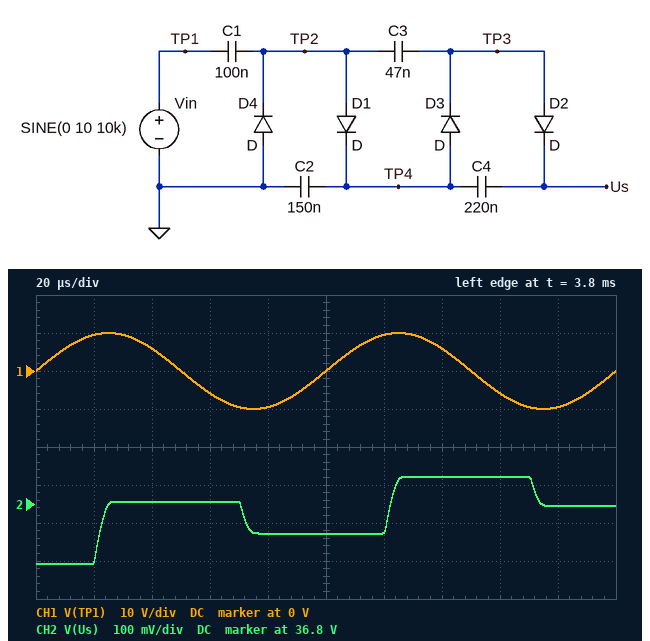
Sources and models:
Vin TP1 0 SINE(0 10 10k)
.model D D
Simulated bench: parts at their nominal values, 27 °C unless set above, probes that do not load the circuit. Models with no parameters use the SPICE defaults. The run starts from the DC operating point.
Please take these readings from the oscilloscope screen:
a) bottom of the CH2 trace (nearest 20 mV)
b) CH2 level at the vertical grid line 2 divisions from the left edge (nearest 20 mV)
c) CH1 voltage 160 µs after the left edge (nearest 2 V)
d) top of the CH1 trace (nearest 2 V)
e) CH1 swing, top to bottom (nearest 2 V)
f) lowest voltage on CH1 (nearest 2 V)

36.64 V
36.80 V
-6 V
10 V
20 V
-10 V
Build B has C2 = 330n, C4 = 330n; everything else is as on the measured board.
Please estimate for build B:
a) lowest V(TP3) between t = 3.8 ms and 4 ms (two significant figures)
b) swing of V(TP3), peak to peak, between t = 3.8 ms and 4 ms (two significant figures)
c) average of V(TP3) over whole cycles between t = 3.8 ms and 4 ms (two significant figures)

17 V
19 V
27 V
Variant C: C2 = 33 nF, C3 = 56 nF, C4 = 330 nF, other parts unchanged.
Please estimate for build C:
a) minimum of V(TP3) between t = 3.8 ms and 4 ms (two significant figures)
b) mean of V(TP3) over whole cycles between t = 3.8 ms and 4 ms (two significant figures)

16 V
25 V
